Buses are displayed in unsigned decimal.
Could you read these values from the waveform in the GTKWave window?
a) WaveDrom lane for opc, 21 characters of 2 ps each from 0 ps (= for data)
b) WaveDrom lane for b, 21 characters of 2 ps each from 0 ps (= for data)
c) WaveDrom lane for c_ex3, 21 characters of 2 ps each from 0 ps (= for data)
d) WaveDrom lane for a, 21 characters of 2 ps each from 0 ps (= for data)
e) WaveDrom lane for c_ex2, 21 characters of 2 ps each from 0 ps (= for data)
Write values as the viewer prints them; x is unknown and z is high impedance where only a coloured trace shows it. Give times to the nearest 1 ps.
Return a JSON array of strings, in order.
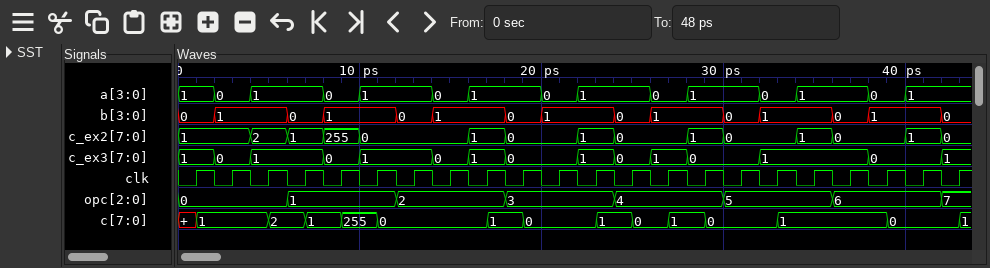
["{name: 'opc', wave: '=..=..=..=..=..=..=..', data: '0 1 2 3 4 5 6'}", "{name: 'b', wave: '==.==.==.==.==.==.==.', data: '0 1 0 1 0 1 0 1 0 1 0 1 0 1'}", "{name: 'c_ex3', wave: '===.==.===.====.=..=.', data: '1 0 1 0 1 0 1 0 1 0 1 0 1 0'}", "{name: 'a', wave: '===.==.==.==.==.==.==', data: '1 0 1 0 1 0 1 0 1 0 1 0 1 0 1'}", "{name: 'c_ex2', wave: '=.====..==.==.==.==.=', data: '1 2 1 255 0 1 0 1 0 1 0 1 0 1'}"]
